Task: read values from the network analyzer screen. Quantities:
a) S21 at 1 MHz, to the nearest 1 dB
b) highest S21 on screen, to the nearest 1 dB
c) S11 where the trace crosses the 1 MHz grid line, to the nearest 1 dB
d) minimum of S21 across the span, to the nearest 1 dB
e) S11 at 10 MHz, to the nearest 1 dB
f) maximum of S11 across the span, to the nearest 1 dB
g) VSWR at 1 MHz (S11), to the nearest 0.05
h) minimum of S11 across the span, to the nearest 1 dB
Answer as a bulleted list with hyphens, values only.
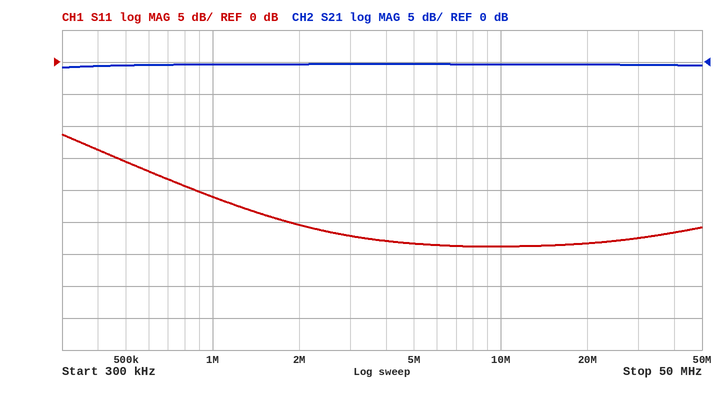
- 0 dB
- 0 dB
- -21 dB
- -1 dB
- -29 dB
- -11 dB
- 1.20
- -29 dB
